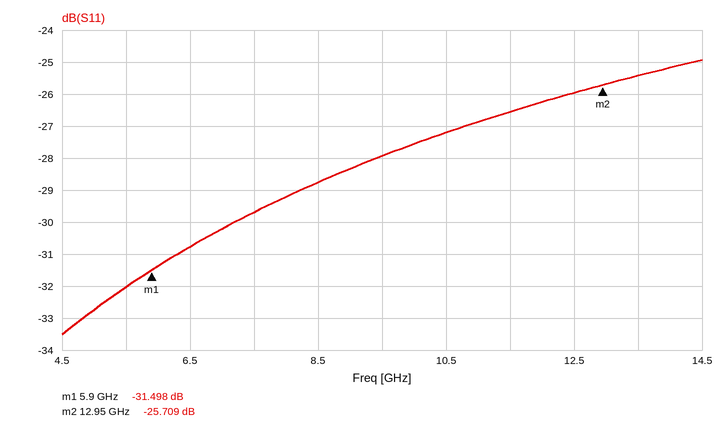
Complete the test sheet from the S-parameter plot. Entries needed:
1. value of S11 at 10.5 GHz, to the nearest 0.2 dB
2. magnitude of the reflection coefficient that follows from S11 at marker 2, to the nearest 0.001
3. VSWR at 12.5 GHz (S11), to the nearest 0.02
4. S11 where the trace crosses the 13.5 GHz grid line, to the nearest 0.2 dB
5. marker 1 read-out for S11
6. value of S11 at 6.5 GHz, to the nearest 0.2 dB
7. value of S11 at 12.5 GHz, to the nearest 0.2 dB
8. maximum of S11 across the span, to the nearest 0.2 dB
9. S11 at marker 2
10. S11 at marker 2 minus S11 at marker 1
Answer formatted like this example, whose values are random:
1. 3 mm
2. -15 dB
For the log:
1. -27.2 dB
2. 0.052
3. 1.10
4. -25.4 dB
5. -31.498 dB
6. -30.8 dB
7. -26.0 dB
8. -25.0 dB
9. -25.709 dB
10. 5.789 dB
